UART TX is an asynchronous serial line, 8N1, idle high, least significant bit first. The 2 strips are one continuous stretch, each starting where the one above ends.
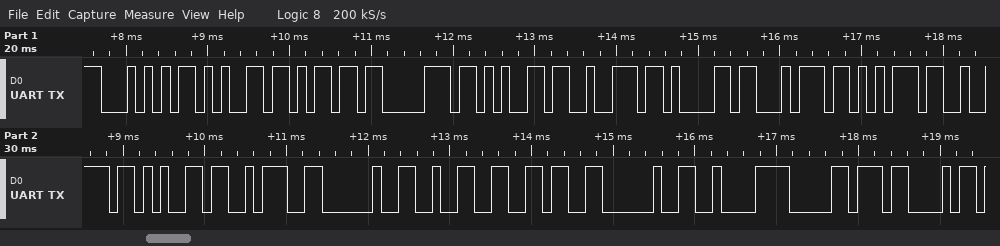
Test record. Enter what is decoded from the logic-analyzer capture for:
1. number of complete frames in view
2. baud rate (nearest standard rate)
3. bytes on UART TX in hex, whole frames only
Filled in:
19
9600 baud
54 65 6D 70 65 72 61 74 75 72 65 3A 20 32 36 20 C2 B0 43
